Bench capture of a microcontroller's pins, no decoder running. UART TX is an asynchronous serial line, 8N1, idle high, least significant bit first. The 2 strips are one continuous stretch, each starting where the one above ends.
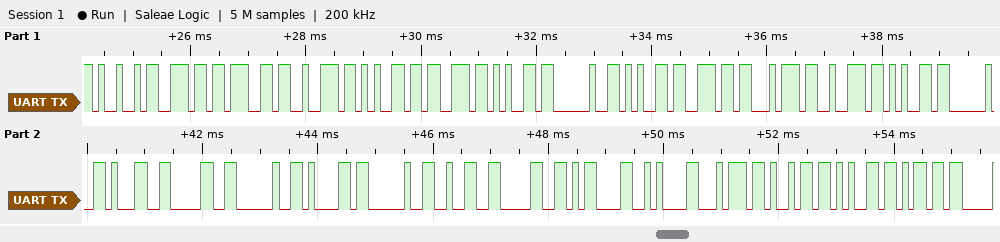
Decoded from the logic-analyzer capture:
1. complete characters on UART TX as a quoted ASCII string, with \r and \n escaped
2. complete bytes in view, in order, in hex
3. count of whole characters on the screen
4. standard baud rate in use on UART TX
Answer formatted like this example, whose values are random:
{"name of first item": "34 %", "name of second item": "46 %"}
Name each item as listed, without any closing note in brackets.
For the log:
{"complete characters on UART TX as a quoted ASCII string, with \\r and \\n escaped": "\"Ingrese entre 10 a 20\\r\\ntiem\"", "complete bytes in view, in order, in hex": "49 6E 67 72 65 73 65 20 65 6E 74 72 65 20 31 30 20 61 20 32 30 0D 0A 74 69 65 6D", "count of whole characters on the screen": "27", "standard baud rate in use on UART TX": "9600 baud"}
